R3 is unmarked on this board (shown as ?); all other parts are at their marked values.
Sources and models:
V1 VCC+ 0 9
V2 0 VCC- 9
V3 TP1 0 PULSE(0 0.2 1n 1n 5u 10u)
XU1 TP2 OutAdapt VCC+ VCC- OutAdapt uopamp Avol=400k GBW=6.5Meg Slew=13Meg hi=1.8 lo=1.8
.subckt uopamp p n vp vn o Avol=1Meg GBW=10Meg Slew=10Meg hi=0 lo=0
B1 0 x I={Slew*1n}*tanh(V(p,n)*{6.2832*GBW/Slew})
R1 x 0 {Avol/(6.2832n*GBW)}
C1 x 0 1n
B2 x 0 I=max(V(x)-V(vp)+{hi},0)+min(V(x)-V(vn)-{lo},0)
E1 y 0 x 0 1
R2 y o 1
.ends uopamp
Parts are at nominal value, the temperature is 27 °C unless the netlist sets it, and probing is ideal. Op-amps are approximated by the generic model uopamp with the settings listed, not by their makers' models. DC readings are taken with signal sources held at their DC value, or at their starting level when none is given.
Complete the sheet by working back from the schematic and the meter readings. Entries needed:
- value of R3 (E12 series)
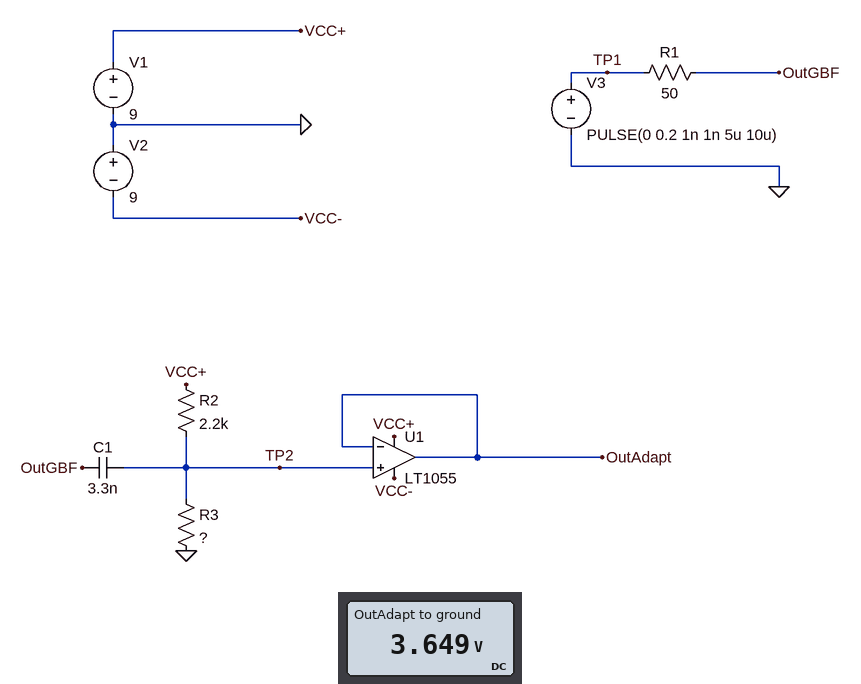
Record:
1.5 kΩ
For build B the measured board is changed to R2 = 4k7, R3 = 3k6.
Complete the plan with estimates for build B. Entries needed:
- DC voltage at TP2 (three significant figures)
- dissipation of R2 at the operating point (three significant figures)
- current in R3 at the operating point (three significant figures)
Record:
3.90 V
5.53 mW
1.08 mA
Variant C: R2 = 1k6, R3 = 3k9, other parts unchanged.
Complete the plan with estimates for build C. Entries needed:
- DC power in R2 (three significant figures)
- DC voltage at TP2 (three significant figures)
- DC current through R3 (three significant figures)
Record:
4.28 mW
6.38 V
1.64 mA
